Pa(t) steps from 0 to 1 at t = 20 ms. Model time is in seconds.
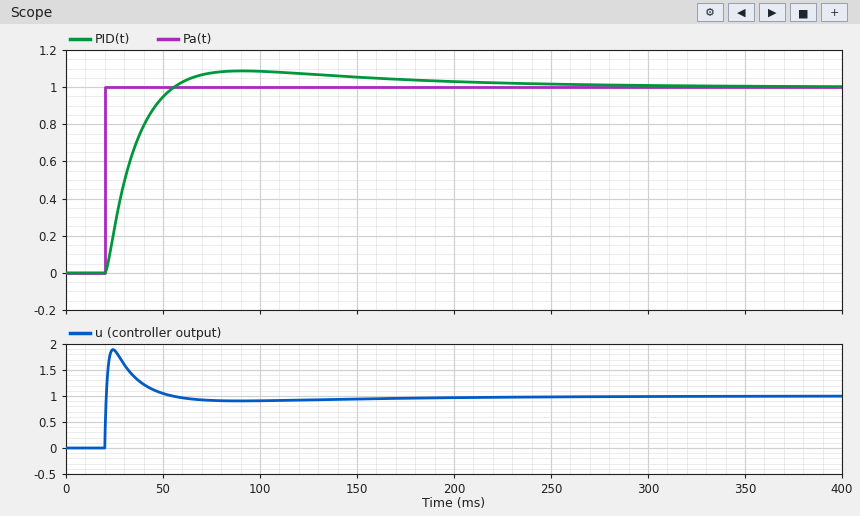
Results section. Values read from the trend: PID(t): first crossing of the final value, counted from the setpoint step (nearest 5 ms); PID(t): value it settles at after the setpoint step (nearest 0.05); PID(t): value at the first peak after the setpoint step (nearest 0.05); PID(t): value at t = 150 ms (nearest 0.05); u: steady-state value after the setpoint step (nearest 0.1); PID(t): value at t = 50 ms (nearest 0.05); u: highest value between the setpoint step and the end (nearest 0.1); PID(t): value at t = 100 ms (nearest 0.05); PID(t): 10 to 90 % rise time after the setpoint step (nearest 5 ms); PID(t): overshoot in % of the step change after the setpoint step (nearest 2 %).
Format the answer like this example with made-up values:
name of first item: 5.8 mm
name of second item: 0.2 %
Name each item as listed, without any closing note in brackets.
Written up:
PID(t): first crossing of the final value, counted from the setpoint step: 35 ms
PID(t): value it settles at after the setpoint step: 1.00
PID(t): value at the first peak after the setpoint step: 1.10
PID(t): value at t = 150 ms: 1.05
u: steady-state value after the setpoint step: 1.0
PID(t): value at t = 50 ms: 0.95
u: highest value between the setpoint step and the end: 1.9
PID(t): value at t = 100 ms: 1.10
PID(t): 10 to 90 % rise time after the setpoint step: 25 ms
PID(t): overshoot in % of the step change after the setpoint step: 8 %
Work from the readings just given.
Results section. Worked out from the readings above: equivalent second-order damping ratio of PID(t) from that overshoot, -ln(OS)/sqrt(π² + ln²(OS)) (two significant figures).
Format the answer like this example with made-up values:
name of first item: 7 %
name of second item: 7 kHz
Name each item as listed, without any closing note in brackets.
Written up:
equivalent second-order damping ratio of PID(t) from that overshoot, -ln(OS)/sqrt(π² + ln²(OS)): 0.63
